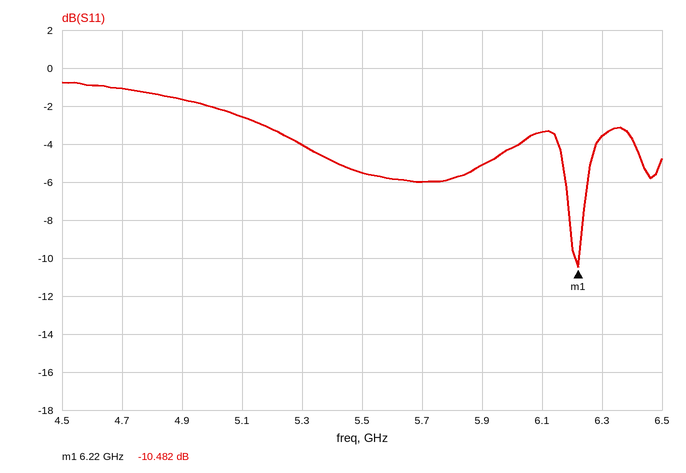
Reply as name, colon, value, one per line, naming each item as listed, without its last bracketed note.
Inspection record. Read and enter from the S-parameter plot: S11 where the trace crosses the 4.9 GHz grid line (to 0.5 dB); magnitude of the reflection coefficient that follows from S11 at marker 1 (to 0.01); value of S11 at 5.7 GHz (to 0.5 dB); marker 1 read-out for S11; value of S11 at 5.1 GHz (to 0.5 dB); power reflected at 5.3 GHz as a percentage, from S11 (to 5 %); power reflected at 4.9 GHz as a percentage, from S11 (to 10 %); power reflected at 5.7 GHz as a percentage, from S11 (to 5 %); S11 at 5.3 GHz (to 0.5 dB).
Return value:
S11 where the trace crosses the 4.9 GHz grid line: -1.5 dB
magnitude of the reflection coefficient that follows from S11 at marker 1: 0.30
value of S11 at 5.7 GHz: -6.0 dB
marker 1 read-out for S11: -10.482 dB
value of S11 at 5.1 GHz: -2.5 dB
power reflected at 5.3 GHz as a percentage, from S11: 40 %
power reflected at 4.9 GHz as a percentage, from S11: 70 %
power reflected at 5.7 GHz as a percentage, from S11: 25 %
S11 at 5.3 GHz: -4.0 dB
